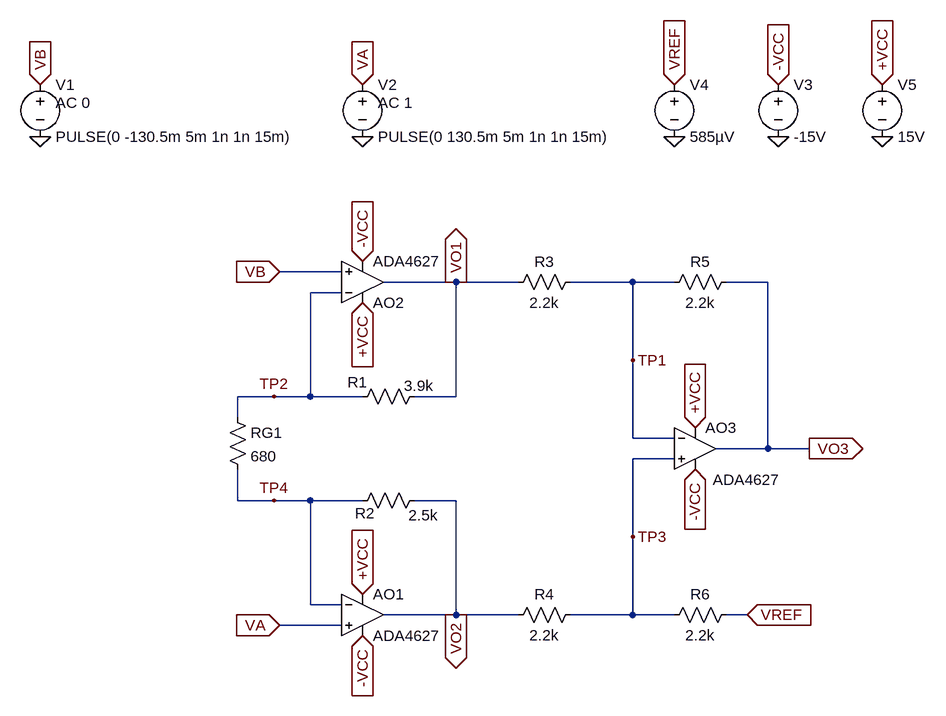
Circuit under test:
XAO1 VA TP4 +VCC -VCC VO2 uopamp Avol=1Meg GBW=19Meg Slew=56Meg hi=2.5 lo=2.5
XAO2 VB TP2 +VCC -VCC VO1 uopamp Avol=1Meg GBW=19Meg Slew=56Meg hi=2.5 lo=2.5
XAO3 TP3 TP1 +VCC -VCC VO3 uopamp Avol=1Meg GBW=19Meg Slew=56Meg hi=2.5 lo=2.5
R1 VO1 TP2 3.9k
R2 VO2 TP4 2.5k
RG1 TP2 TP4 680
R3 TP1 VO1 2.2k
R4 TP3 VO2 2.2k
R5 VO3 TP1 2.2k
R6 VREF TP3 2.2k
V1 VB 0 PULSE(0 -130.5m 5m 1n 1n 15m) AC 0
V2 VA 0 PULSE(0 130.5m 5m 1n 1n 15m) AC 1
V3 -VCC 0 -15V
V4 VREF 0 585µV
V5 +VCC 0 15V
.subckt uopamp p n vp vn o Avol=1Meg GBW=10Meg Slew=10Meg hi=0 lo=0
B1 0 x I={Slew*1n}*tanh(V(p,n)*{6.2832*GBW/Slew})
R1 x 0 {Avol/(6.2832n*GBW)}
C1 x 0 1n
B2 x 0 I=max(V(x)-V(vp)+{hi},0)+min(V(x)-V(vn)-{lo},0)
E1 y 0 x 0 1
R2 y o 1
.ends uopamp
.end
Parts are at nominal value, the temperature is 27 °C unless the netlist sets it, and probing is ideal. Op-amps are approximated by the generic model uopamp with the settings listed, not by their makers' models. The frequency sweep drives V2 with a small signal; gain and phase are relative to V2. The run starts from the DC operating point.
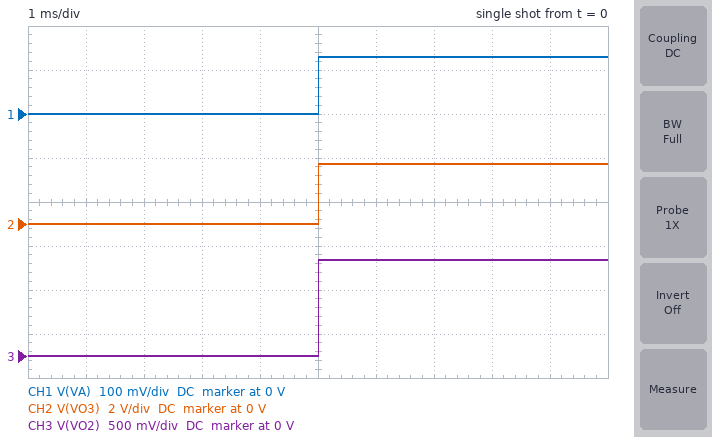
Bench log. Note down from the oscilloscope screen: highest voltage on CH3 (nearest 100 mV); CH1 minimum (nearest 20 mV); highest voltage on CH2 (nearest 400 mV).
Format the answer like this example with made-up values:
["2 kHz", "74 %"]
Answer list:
["1.1 V", "0 V", "2.8 V"]
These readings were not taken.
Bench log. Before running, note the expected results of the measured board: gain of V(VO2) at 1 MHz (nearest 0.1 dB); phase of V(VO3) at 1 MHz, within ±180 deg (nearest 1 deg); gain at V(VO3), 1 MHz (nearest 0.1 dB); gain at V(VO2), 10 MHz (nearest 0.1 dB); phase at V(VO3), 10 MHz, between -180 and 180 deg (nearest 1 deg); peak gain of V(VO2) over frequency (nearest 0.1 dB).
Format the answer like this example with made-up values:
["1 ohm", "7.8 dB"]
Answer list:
["12.3 dB", "-35 deg", "19.2 dB", "1.2 dB", "-126 deg", "13.4 dB"]
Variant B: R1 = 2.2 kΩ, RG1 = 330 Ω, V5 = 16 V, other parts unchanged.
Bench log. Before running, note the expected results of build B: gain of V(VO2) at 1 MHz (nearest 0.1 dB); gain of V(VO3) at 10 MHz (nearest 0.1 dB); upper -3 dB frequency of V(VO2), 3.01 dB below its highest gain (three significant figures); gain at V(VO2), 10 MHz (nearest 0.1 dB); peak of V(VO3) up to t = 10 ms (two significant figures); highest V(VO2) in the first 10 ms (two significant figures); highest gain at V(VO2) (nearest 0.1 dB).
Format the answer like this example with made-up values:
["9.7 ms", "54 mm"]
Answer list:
["16.5 dB", "2.3 dB", "1.26 MHz", "2.2 dB", "4.0 V", "2.1 V", "18.7 dB"]
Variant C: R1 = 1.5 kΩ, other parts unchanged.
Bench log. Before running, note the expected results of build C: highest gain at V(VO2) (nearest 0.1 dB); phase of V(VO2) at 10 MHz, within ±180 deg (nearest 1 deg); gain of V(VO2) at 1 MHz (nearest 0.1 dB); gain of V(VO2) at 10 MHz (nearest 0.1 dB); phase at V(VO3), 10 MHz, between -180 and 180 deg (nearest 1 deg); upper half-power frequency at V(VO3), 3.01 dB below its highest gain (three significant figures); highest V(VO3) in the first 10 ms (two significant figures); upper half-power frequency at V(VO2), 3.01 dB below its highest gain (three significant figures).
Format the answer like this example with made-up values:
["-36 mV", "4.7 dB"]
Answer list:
["13.4 dB", "-65 deg", "12.9 dB", "2.9 dB", "-121 deg", "2.56 MHz", "1.8 V", "2.83 MHz"]
